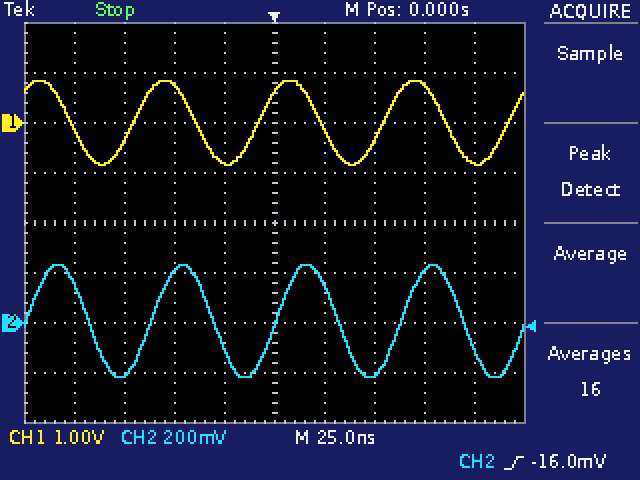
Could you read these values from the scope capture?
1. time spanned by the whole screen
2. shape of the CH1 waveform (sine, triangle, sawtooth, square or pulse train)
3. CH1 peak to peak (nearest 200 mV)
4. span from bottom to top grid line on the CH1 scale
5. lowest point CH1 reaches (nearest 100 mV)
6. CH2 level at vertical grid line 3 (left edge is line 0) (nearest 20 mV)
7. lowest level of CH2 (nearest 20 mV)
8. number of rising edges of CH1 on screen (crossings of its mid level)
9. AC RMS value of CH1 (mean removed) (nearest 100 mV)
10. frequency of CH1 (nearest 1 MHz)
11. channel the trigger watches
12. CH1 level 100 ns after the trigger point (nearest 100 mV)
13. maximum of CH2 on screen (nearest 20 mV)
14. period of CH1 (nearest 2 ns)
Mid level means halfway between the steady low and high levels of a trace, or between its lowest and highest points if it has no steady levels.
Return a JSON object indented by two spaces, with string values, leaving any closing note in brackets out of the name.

{
  "time spanned by the whole screen": "250 ns",
  "shape of the CH1 waveform": "sine",
  "CH1 peak to peak": "1.6 V",
  "span from bottom to top grid line on the CH1 scale": "8 V",
  "lowest point CH1 reaches": "-800 mV",
  "CH2 level at vertical grid line 3 (left edge is line 0)": "200 mV",
  "lowest level of CH2": "-220 mV",
  "number of rising edges of CH1 on screen": "4",
  "AC RMS value of CH1 (mean removed)": "600 mV",
  "frequency of CH1": "16 MHz",
  "channel the trigger watches": "CH2",
  "CH1 level 100 ns after the trigger point": "-800 mV",
  "maximum of CH2 on screen": "240 mV",
  "period of CH1": "62 ns"
}
